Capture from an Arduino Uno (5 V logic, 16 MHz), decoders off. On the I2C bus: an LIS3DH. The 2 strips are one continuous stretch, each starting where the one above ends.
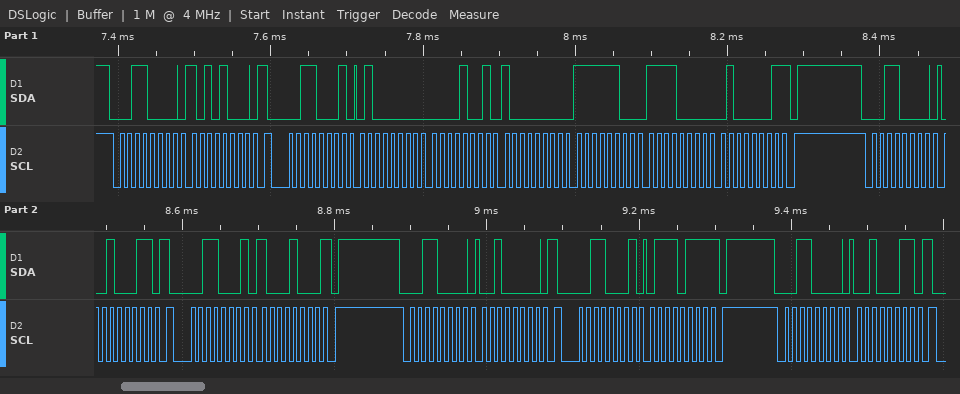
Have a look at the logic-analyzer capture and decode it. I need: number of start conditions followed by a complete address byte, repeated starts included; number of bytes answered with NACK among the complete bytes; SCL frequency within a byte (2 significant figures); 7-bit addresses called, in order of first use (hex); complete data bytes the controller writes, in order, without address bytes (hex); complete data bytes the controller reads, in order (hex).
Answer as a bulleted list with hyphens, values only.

- 7
- 3
- 100 kHz
- 0x18
- A8 23 20 23
- 40 09 80 FC F0 41 88 77
